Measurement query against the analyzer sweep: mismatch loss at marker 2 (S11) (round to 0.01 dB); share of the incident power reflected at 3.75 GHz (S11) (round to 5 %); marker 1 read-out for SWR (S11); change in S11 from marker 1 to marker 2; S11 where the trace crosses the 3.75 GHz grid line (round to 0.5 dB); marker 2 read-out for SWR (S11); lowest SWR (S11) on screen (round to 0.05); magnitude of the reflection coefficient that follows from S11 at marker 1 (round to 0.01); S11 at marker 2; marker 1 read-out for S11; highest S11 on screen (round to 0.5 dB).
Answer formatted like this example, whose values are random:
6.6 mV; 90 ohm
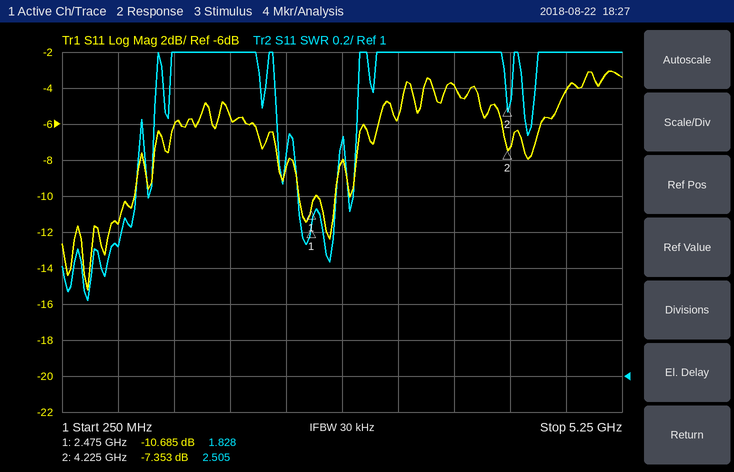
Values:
0.88 dB; 40 %; 1.828; 3.332 dB; -4.0 dB; 2.505; 1.40; 0.29; -7.353 dB; -10.685 dB; -3.0 dB
